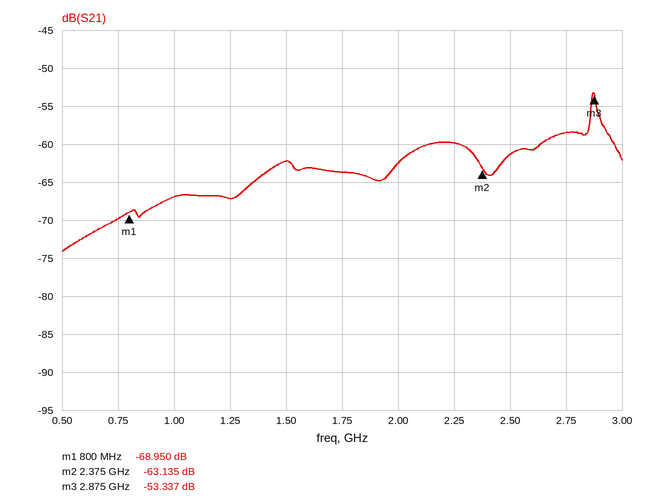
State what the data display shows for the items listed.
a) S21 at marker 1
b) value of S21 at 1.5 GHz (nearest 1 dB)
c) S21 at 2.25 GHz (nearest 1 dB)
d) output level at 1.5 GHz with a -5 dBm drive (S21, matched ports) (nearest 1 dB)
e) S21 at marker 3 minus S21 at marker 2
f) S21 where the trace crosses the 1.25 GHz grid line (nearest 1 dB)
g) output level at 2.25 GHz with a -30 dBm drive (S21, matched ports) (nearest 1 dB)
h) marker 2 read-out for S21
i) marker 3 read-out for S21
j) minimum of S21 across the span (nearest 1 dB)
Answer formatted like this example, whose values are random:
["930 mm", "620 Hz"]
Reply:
["-68.950 dB", "-62 dB", "-60 dB", "-67 dBm", "9.798 dB", "-67 dB", "-90 dBm", "-63.135 dB", "-53.337 dB", "-74 dB"]
